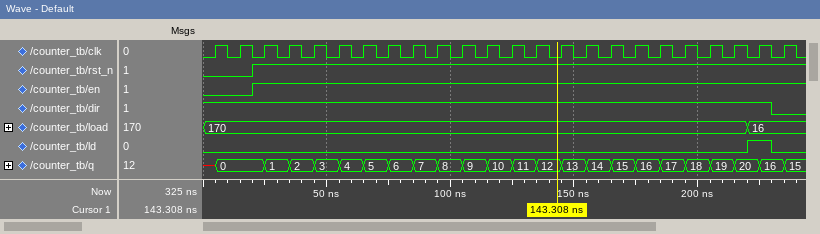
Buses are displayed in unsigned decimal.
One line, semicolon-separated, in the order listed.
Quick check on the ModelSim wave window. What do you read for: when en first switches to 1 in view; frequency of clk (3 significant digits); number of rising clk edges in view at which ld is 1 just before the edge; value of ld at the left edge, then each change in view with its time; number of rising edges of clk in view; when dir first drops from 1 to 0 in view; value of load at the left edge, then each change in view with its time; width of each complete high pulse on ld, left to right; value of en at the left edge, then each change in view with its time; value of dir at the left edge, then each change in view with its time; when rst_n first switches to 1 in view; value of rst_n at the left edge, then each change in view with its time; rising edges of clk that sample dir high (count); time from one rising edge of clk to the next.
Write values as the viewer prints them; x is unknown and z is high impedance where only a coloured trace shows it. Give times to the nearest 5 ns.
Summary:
20 ns; 100 MHz; 1; 0, 1 at 220 ns, 0 at 230 ns; 24; 230 ns; 170, 16 at 220 ns; 10 ns; 0, 1 at 20 ns; 1, 0 at 230 ns; 20 ns; 0, 1 at 20 ns; 23; 10 ns
